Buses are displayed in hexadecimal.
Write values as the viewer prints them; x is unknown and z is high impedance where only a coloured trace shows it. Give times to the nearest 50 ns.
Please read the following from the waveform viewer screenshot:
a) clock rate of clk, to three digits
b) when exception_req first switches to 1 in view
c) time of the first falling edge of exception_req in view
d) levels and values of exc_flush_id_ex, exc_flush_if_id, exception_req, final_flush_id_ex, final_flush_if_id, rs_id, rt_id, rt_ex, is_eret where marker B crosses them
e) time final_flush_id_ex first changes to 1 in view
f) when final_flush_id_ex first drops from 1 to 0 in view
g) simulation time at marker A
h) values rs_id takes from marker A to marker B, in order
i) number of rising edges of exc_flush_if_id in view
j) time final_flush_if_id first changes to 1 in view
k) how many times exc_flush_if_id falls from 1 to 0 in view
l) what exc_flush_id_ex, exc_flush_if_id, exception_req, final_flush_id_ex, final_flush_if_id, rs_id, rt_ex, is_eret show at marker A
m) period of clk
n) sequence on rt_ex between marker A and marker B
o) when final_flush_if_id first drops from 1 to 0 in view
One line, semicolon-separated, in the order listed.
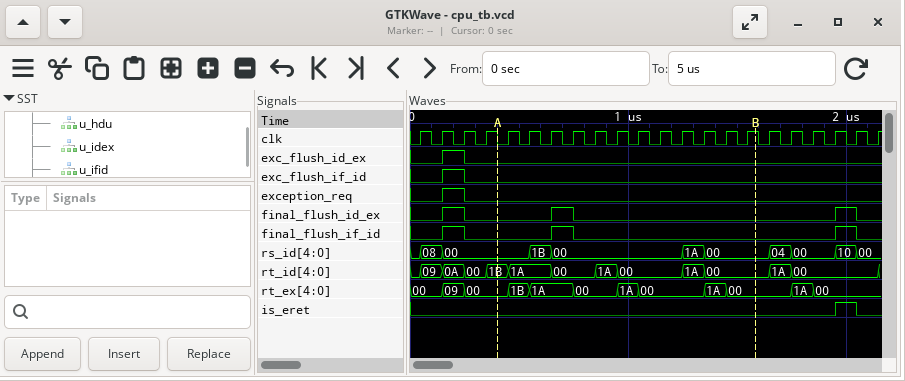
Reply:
10.0 MHz; 150 ns; 250 ns; exc_flush_id_ex=0, exc_flush_if_id=0, exception_req=0, final_flush_id_ex=0, final_flush_if_id=0, rs_id=00, rt_id=00, rt_ex=00, is_eret=0; 150 ns; 250 ns; 400 ns; 00, 1B, 00, 1A, 00; 1; 150 ns; 1; exc_flush_id_ex=0, exc_flush_if_id=0, exception_req=0, final_flush_id_ex=0, final_flush_if_id=0, rs_id=00, rt_ex=00, is_eret=0; 100 ns; 00, 1B, 1A, 00, 1A, 00, 1A, 00; 250 ns
